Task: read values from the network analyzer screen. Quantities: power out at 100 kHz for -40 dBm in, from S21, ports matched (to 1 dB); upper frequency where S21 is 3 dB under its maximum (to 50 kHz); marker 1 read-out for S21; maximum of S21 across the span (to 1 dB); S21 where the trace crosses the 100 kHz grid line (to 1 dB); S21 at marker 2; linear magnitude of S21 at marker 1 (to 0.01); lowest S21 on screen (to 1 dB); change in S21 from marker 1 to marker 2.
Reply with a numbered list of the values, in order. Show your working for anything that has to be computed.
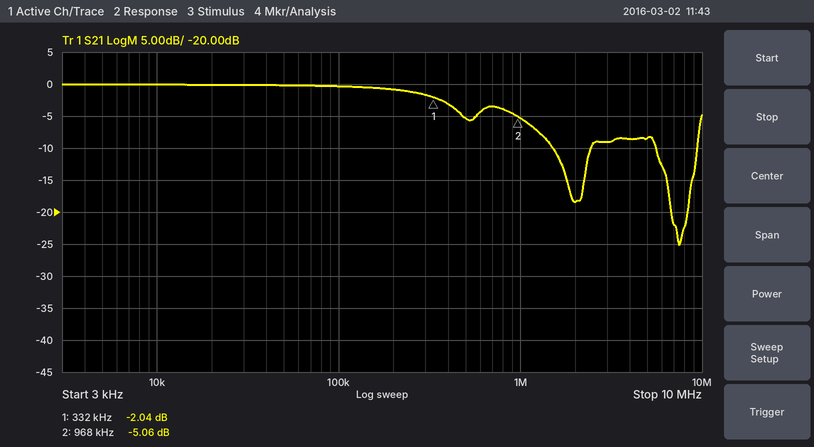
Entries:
1. -40 dBm + (0 dB) = -40 dBm
2. 400 kHz
3. -2.04 dB
4. 0 dB
5. 0 dB
6. -5.06 dB
7. 10^(-2.04/20) ≈ 0.79
8. -25 dB
9. -5.06 − (-2.04) = -3.02 dB
